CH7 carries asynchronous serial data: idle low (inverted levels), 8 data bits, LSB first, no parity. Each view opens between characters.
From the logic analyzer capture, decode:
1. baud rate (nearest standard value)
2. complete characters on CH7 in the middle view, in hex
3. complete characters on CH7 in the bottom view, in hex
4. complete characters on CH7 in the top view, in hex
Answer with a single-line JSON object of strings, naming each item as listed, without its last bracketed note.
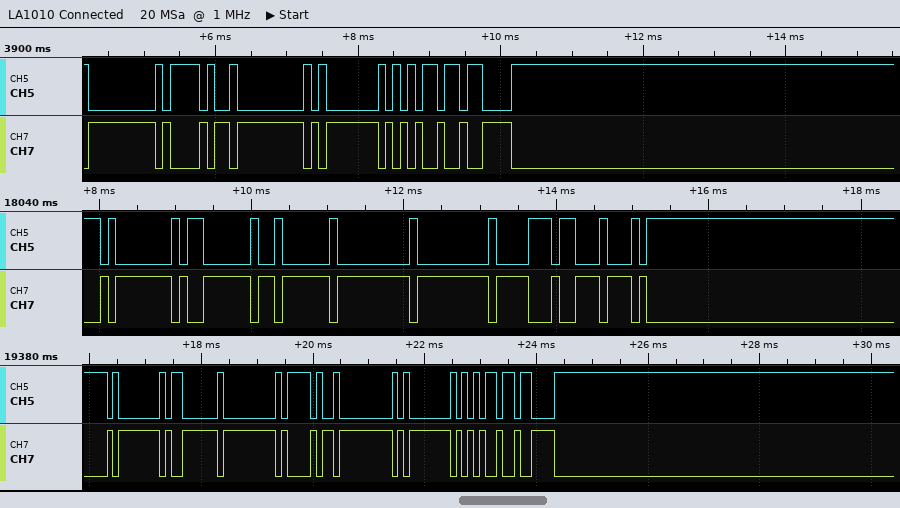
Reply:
{"baud rate": "9600 baud", "complete characters on CH7 in the middle view, in hex": "01, 03, 02, 00, 00, B8, 44", "complete characters on CH7 in the bottom view, in hex": "01, 03, 00, 2F, 00, 01, B5, C3", "complete characters on CH7 in the top view, in hex": "00, 2F, 00, 01, B5, C3"}
